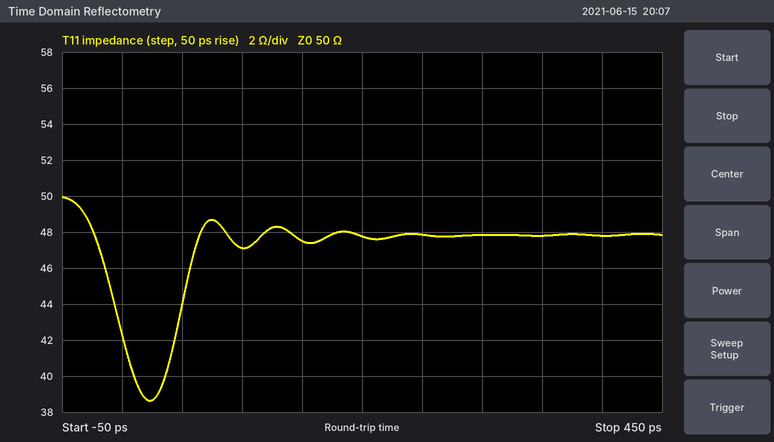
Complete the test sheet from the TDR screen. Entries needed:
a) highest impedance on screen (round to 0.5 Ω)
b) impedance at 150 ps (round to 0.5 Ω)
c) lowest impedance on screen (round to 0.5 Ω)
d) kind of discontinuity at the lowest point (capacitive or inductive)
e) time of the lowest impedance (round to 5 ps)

50.0 Ω
47.5 Ω
38.5 Ω
capacitive
25 ps
